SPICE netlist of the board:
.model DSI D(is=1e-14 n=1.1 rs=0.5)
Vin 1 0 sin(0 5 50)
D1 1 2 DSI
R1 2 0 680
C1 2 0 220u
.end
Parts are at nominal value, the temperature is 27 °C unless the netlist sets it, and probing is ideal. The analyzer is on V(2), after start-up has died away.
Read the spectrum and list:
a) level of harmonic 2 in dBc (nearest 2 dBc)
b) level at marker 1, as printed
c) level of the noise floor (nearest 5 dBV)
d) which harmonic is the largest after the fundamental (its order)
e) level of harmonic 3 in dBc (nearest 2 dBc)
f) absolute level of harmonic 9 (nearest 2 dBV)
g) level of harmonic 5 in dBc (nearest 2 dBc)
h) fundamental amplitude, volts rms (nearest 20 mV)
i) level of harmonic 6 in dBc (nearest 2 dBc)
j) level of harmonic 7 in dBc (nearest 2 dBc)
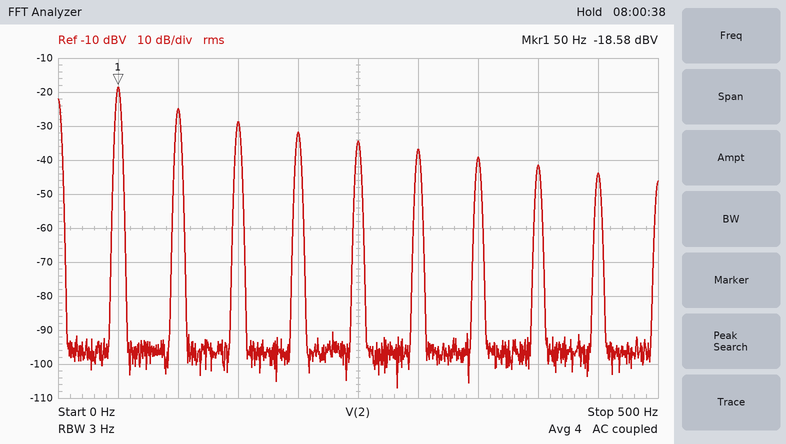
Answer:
-6 dBc
-18.58 dBV
-95 dBV
2
-10 dBc
-44 dBV
-16 dBc
120 mV
-18 dBc
-20 dBc
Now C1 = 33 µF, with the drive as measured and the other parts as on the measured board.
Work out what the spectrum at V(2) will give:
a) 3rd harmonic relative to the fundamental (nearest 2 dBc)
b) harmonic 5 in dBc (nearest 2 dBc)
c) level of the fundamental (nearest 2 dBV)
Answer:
-12 dBc
-22 dBc
-4 dBV
